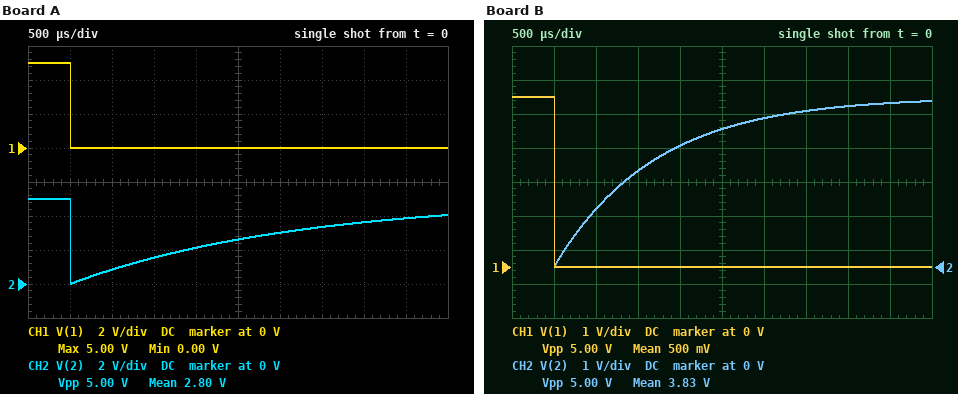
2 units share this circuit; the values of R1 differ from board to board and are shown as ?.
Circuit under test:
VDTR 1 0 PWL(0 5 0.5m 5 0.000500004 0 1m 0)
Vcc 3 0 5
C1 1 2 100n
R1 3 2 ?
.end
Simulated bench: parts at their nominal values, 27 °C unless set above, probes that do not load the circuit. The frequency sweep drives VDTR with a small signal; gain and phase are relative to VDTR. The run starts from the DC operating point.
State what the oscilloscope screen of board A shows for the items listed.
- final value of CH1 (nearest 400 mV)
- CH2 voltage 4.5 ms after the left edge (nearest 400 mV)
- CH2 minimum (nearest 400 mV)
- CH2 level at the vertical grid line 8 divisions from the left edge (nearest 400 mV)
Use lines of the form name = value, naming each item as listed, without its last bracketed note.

final value of CH1 = 0 V
CH2 voltage 4.5 ms after the left edge = 4.0 V
CH2 minimum = 0 V
CH2 level at the vertical grid line 8 divisions from the left edge = 3.6 V
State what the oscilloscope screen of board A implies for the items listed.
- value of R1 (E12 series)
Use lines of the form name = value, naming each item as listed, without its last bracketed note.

value of R1 = 27 kΩ
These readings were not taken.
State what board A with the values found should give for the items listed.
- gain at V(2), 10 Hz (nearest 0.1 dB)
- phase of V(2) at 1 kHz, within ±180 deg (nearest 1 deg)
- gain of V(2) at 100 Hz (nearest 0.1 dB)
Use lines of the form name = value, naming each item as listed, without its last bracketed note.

gain at V(2), 10 Hz = -15.5 dB
phase of V(2) at 1 kHz, within ±180 deg = 3 deg
gain of V(2) at 100 Hz = -1.3 dB
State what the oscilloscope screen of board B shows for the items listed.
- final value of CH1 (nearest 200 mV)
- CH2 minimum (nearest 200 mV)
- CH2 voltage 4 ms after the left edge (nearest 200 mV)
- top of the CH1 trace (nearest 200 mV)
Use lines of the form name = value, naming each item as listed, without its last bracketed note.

final value of CH1 = 0 V
CH2 minimum = 0 V
CH2 voltage 4 ms after the left edge = 4.8 V
top of the CH1 trace = 5.0 V
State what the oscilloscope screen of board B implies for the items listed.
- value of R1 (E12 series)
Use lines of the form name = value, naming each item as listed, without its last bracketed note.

value of R1 = 12 kΩ
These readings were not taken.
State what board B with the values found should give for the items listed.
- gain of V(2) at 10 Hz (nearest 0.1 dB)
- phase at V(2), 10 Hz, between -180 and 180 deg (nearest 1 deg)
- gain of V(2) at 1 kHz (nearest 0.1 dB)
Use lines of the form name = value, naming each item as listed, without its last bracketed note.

gain of V(2) at 10 Hz = -22.5 dB
phase at V(2), 10 Hz, between -180 and 180 deg = 86 deg
gain of V(2) at 1 kHz = -0.1 dB
